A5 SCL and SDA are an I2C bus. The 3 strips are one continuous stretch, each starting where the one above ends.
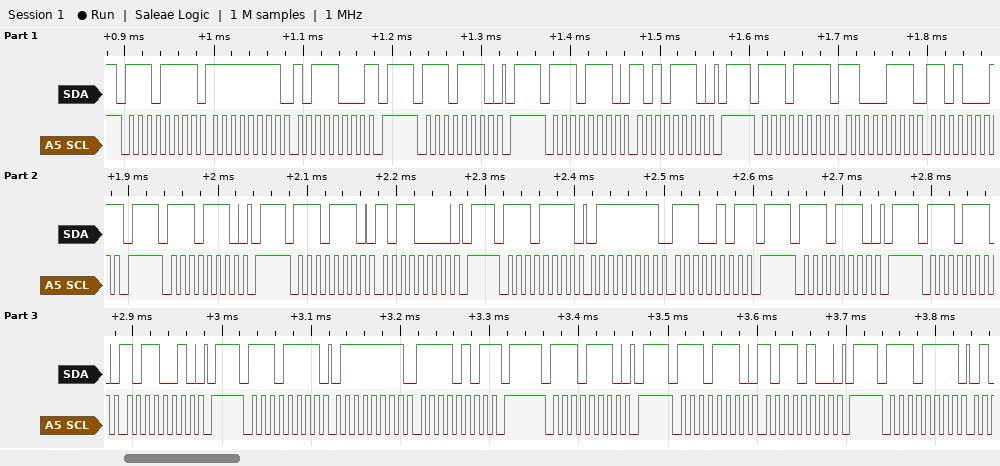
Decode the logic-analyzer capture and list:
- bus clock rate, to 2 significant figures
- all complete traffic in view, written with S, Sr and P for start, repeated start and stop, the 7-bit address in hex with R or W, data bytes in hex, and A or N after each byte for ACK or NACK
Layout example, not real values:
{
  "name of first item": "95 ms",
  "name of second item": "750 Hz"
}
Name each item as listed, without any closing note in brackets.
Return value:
{
  "bus clock rate, to 2 significant figures": "100 kHz",
  "all complete traffic in view, written with S, Sr and P for start, repeated start and stop, the 7-bit address in hex with R or W, data bytes in hex, and A or N after each byte for ACK or NACK": "S 77R A FF A B8 N P S 77W A P S 77W A AE A P S 77R A C7 A D1 N P S 77W A P S 77W A B0 A P S 77R A 7F A E5 N P S 77W A P S 77W A B2 A P S 77R A 7F A F5 N P S 77W A P S 77W A B4 A P S 77R A"
}
